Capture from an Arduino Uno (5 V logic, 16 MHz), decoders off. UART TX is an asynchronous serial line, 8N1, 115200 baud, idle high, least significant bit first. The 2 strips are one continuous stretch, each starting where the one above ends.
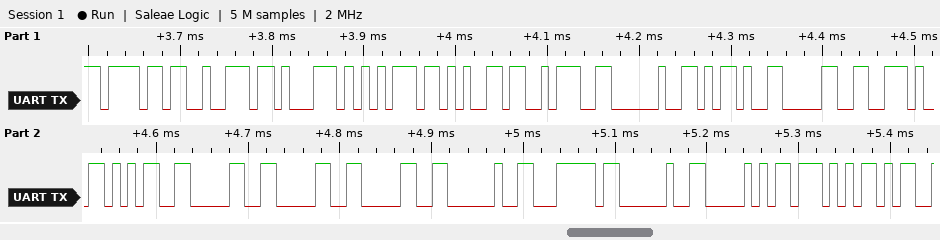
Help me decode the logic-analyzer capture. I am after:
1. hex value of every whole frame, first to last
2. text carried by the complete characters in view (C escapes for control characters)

6F 72 71 75 65 3A 20 2D 30 2E 35 30 30 30 20 7C 20 50 57
"orque: -0.5000 | PW"
